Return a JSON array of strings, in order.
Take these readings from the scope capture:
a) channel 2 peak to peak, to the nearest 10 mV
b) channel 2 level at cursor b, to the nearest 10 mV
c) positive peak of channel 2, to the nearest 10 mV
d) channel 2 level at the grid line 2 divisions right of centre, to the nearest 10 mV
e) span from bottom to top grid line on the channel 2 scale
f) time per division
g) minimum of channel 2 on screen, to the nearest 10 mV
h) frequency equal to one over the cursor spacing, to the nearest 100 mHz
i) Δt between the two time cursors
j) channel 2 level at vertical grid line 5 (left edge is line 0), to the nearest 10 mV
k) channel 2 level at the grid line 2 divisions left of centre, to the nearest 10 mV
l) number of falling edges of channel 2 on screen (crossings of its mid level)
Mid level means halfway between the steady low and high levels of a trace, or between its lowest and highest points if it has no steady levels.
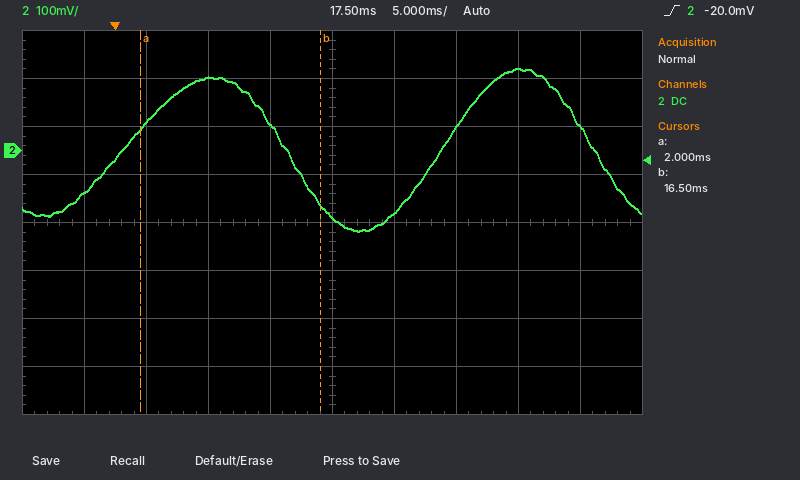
["340 mV", "-110 mV", "170 mV", "50 mV", "800 mV", "5 ms", "-170 mV", "69.0 Hz", "14.5 ms", "-140 mV", "150 mV", "2"]
